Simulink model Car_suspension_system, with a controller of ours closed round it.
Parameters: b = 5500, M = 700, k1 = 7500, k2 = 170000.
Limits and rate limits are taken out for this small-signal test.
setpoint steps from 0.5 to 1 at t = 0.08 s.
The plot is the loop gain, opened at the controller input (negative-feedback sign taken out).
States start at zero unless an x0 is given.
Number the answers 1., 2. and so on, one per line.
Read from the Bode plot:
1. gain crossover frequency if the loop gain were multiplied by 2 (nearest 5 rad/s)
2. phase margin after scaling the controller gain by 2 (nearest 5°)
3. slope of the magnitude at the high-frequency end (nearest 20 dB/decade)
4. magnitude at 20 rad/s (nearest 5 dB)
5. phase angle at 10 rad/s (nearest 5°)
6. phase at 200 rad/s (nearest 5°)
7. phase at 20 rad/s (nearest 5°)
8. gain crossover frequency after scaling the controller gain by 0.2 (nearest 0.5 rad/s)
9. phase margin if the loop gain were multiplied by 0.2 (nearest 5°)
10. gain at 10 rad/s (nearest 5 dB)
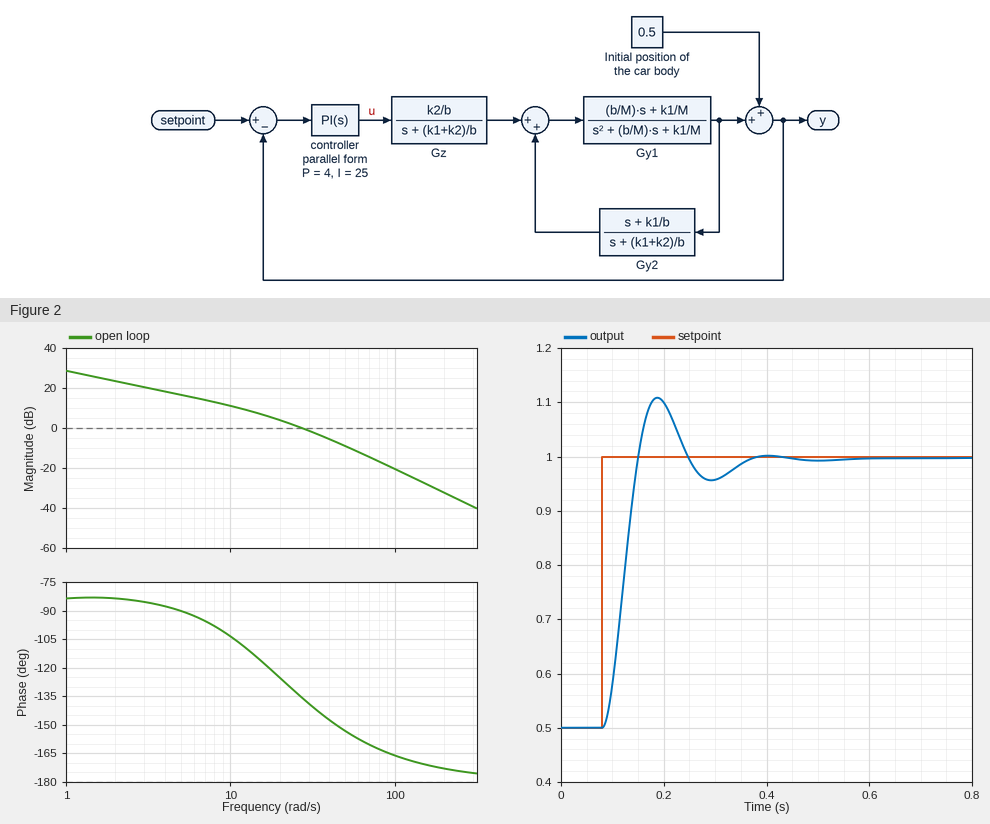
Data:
1. 40 rad/s
2. 30°
3. -40 dB/decade
4. 5 dB
5. -105°
6. -175°
7. -125°
8. 7.0 rad/s
9. 85°
10. 10 dB
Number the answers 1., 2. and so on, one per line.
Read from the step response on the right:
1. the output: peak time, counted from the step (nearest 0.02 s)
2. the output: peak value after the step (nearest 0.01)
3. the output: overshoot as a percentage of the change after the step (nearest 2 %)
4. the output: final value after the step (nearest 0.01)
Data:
1. 0.10 s
2. 1.11
3. 22 %
4. 1.00
